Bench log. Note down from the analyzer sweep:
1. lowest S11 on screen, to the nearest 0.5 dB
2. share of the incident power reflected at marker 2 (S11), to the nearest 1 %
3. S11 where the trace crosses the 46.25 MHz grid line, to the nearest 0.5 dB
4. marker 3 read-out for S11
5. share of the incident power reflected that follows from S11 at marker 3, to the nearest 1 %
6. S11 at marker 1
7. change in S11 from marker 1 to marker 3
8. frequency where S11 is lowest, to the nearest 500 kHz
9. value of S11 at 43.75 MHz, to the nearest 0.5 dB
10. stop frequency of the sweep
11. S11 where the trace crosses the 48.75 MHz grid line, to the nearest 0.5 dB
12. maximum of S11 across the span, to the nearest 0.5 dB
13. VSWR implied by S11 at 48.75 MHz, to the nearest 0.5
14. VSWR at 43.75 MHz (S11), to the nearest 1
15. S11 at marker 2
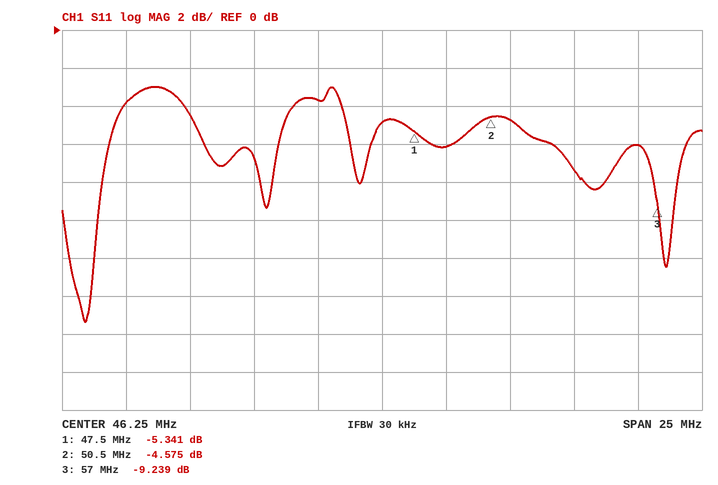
-15.5 dB
35 %
-5.0 dB
-9.239 dB
12 %
-5.341 dB
-3.898 dB
34.5 MHz
-3.5 dB
58.75 MHz
-6.0 dB
-3.0 dB
3.0
5
-4.575 dB
